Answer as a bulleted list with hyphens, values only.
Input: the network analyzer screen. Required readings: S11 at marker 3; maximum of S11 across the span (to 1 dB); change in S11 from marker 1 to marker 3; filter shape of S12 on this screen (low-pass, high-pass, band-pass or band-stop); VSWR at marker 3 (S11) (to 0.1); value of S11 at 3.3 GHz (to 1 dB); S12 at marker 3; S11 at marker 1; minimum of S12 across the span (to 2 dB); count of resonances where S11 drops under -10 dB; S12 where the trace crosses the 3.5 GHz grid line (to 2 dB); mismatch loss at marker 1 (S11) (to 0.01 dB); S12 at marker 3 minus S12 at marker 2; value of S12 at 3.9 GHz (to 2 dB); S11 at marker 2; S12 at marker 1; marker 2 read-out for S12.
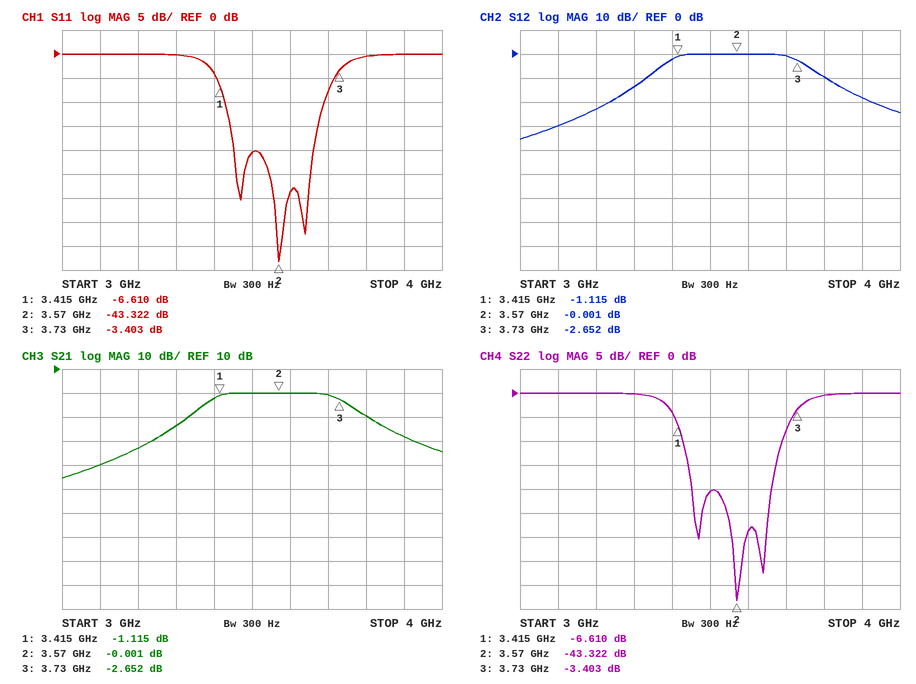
- -3.403 dB
- 0 dB
- 3.207 dB
- band-pass
- 5.2
- 0 dB
- -2.652 dB
- -6.610 dB
- -36 dB
- 3
- 0 dB
- 1.07 dB
- -2.651 dB
- -18 dB
- -43.322 dB
- -1.115 dB
- -0.001 dB
